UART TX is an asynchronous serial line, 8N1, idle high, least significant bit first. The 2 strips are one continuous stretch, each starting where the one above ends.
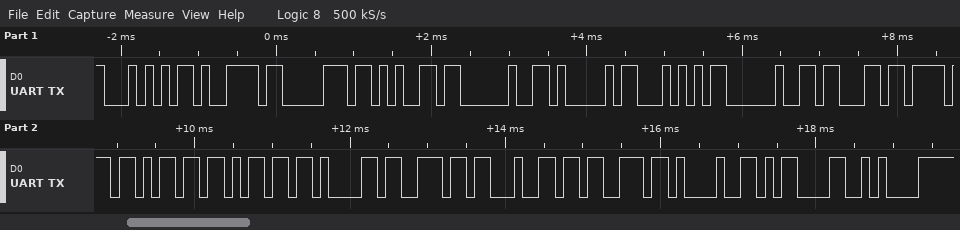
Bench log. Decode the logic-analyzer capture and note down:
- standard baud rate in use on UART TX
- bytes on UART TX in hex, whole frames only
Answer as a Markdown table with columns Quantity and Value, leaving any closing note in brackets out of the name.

| Quantity | Value |
|---|---|
| standard baud rate in use on UART TX | 9600 baud |
| bytes on UART TX in hex, whole frames only | 0x54 0x79 0x70 0x65 0x20 0x41 0x54 0x20 0x63 0x6F 0x6D 0x6D 0x61 0x6E 0x64 0x73 0x21 0x0D 0x0A |
